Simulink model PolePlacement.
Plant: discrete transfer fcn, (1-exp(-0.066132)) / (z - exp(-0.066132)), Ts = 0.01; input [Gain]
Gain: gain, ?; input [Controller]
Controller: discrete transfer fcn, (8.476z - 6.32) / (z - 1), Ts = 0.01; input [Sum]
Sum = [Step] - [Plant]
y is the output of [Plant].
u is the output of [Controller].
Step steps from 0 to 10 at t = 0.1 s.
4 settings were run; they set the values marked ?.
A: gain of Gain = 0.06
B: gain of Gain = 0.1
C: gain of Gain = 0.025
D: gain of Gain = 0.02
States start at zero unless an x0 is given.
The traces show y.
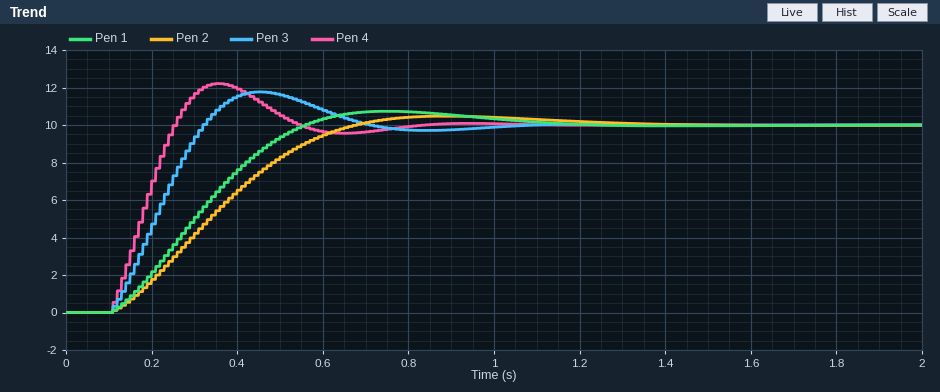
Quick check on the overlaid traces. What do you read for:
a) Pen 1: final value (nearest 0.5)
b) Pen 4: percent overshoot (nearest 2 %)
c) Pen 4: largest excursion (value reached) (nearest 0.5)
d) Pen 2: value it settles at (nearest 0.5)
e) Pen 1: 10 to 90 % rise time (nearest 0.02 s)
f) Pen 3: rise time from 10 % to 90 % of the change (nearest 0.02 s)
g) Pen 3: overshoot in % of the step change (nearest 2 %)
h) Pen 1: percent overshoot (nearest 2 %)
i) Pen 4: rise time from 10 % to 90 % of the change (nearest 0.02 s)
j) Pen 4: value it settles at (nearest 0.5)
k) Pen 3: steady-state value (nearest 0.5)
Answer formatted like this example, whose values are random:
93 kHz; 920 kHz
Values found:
10.0; 22 %; 12.0; 10.0; 0.32 s; 0.16 s; 18 %; 8 %; 0.12 s; 10.0; 10.0
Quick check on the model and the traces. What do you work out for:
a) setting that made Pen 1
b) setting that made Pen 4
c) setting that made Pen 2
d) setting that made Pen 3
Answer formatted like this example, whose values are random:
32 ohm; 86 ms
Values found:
C; B; D; A
